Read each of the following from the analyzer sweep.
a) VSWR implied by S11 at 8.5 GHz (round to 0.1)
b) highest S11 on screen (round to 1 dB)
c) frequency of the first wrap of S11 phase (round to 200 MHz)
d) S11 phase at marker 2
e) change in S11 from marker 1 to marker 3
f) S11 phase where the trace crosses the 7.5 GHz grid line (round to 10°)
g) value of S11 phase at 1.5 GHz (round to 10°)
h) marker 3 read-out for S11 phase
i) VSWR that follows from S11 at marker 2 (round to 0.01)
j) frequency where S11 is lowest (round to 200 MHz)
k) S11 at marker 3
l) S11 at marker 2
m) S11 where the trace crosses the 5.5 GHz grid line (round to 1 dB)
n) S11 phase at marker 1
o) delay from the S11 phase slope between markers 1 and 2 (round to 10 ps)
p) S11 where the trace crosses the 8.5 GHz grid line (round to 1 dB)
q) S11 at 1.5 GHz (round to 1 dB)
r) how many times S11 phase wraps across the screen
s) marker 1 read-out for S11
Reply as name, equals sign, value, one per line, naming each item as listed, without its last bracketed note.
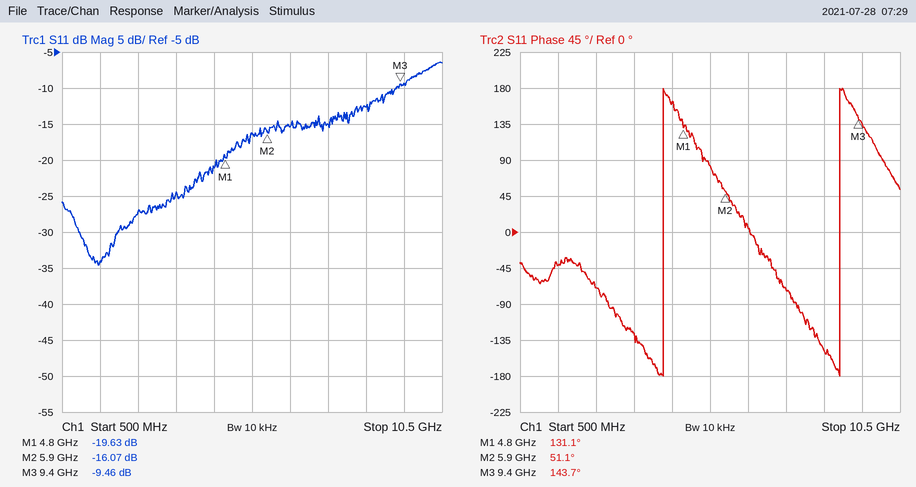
VSWR implied by S11 at 8.5 GHz = 1.6
highest S11 on screen = -6 dB
frequency of the first wrap of S11 phase = 4.2 GHz
S11 phase at marker 2 = 51.1°
change in S11 from marker 1 to marker 3 = 10.17 dB
S11 phase where the trace crosses the 7.5 GHz grid line = -70°
value of S11 phase at 1.5 GHz = -40°
marker 3 read-out for S11 phase = 143.7°
VSWR that follows from S11 at marker 2 = 1.37
frequency where S11 is lowest = 1.4 GHz
S11 at marker 3 = -9.46 dB
S11 at marker 2 = -16.07 dB
S11 where the trace crosses the 5.5 GHz grid line = -16 dB
S11 phase at marker 1 = 131.1°
delay from the S11 phase slope between markers 1 and 2 = 200 ps
S11 where the trace crosses the 8.5 GHz grid line = -13 dB
S11 at 1.5 GHz = -34 dB
how many times S11 phase wraps across the screen = 2
marker 1 read-out for S11 = -19.63 dB
